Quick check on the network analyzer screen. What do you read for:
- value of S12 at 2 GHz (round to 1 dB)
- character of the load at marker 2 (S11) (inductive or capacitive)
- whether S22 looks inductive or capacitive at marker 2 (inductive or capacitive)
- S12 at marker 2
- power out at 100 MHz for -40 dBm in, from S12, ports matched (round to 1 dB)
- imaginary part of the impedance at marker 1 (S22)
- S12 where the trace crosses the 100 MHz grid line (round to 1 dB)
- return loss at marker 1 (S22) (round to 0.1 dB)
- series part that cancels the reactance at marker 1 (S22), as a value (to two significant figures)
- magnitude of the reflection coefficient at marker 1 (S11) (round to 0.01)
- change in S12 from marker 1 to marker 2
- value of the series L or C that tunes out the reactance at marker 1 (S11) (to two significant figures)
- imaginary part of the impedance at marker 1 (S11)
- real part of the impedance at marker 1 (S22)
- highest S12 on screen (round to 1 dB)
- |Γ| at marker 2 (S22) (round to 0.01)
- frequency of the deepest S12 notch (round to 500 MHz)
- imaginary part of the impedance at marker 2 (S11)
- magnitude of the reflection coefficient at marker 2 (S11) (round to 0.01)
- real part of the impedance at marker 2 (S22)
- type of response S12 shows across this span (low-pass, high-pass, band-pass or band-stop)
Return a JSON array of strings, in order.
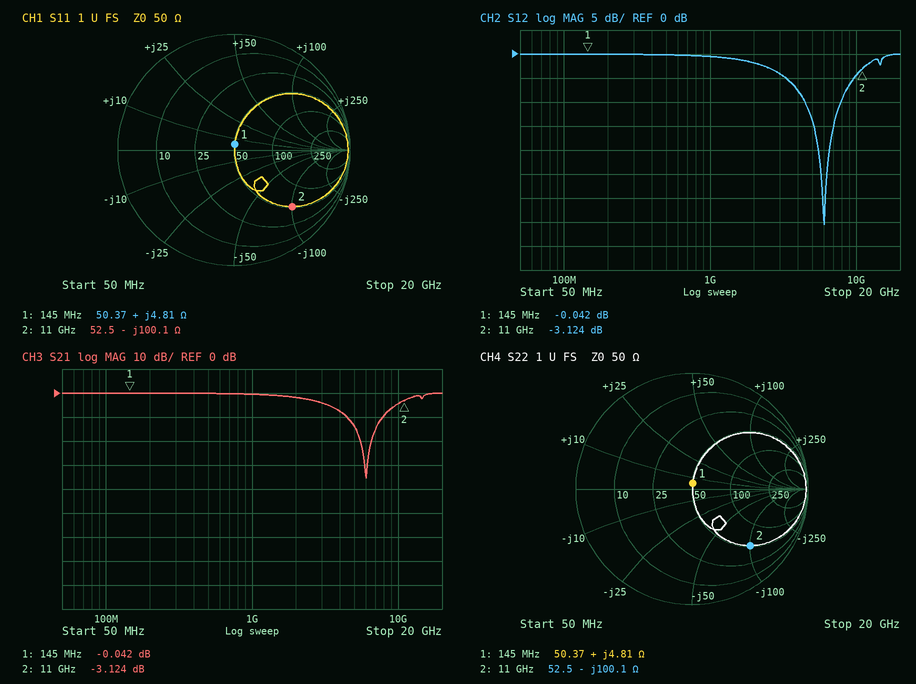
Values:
["-2 dB", "capacitive", "capacitive", "-3.124 dB", "-40 dBm", "+4.81 Ω", "0 dB", "26.4 dB", "230 pF", "0.05", "-3.082 dB", "230 pF", "+4.81 Ω", "50.37 Ω", "0 dB", "0.70", "6.0 GHz", "-100.1 Ω", "0.70", "52.5 Ω", "band-stop"]
